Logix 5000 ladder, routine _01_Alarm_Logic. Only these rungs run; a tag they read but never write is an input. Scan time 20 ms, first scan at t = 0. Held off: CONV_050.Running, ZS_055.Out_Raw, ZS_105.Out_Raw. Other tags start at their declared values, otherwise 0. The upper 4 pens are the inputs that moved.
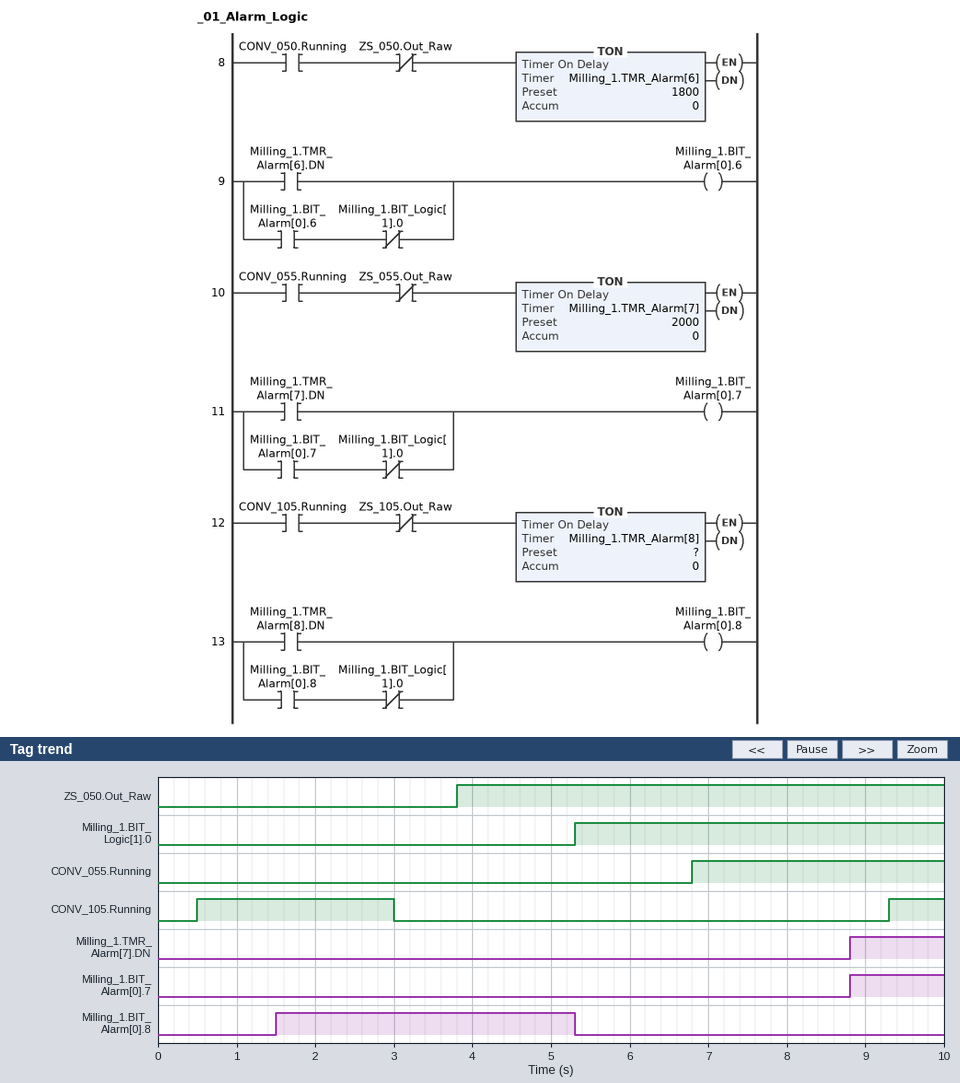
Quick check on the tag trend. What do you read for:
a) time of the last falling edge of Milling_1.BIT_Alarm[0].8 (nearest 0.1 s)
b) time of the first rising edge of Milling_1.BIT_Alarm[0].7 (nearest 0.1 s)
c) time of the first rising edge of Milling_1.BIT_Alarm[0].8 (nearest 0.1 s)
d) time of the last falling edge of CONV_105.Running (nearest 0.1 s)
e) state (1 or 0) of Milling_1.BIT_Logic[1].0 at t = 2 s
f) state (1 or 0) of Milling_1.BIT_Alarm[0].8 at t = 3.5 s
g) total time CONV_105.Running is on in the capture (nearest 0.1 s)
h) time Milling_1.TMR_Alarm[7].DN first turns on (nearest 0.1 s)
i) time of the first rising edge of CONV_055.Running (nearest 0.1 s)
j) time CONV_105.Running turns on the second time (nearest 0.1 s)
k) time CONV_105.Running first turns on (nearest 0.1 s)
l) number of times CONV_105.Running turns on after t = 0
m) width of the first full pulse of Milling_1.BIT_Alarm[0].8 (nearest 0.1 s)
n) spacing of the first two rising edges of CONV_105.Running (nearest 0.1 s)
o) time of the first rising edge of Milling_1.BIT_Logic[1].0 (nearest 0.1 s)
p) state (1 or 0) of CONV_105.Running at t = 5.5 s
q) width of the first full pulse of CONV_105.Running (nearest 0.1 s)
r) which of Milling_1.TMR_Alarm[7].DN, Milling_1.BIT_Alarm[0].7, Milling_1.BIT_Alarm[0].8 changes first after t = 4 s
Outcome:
5.3 s
8.8 s
1.5 s
3.0 s
0
1
3.2 s
8.8 s
6.8 s
9.3 s
0.5 s
2
3.8 s
8.8 s
5.3 s
0
2.5 s
Milling_1.BIT_Alarm[0].8
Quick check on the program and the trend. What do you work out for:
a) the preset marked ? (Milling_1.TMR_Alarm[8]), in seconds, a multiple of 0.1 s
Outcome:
1.0 s
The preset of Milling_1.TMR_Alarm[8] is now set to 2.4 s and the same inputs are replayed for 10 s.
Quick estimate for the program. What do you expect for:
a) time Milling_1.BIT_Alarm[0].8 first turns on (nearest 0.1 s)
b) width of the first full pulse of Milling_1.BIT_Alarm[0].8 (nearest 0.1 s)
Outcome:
2.9 s
2.4 s
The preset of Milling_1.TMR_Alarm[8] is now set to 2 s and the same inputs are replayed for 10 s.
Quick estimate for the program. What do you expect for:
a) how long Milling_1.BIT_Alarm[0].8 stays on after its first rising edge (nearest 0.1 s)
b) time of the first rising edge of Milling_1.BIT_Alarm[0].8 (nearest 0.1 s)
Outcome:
2.8 s
2.5 s
